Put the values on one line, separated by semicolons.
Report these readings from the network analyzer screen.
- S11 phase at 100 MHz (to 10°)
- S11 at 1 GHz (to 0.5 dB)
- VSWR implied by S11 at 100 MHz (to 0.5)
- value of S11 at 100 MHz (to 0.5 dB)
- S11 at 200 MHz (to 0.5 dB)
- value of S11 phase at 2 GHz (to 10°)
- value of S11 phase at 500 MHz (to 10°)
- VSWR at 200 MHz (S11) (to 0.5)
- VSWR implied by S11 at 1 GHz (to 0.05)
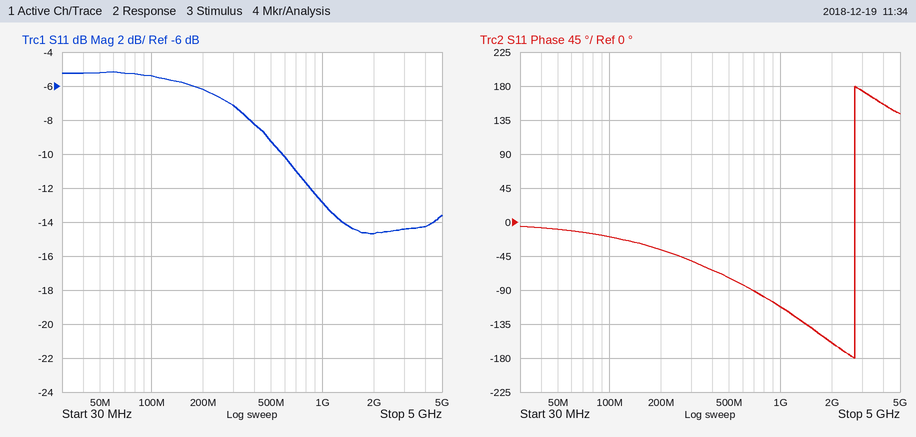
-20°; -13.0 dB; 3.5; -5.5 dB; -6.0 dB; -160°; -70°; 3.0; 1.60
